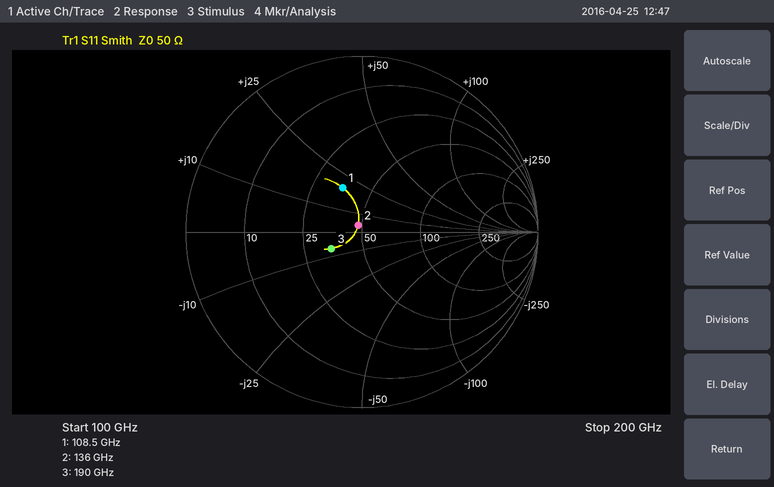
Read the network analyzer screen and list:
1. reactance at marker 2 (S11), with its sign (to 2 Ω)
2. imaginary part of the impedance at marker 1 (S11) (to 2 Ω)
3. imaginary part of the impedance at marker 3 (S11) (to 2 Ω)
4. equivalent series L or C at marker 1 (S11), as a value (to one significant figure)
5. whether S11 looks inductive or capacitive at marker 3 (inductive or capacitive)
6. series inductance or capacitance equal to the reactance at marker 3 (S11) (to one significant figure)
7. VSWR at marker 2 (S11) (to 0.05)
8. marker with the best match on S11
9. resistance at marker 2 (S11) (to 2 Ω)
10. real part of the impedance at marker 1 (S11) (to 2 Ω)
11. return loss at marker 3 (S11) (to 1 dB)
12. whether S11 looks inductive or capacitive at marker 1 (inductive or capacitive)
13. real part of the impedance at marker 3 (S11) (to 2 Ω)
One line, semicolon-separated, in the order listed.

+4 Ω; +20 Ω; -6 Ω; 30 pH; capacitive; 100 fF; 1.10; marker 2; 48 Ω; 36 Ω; 14 dB; inductive; 34 Ω
